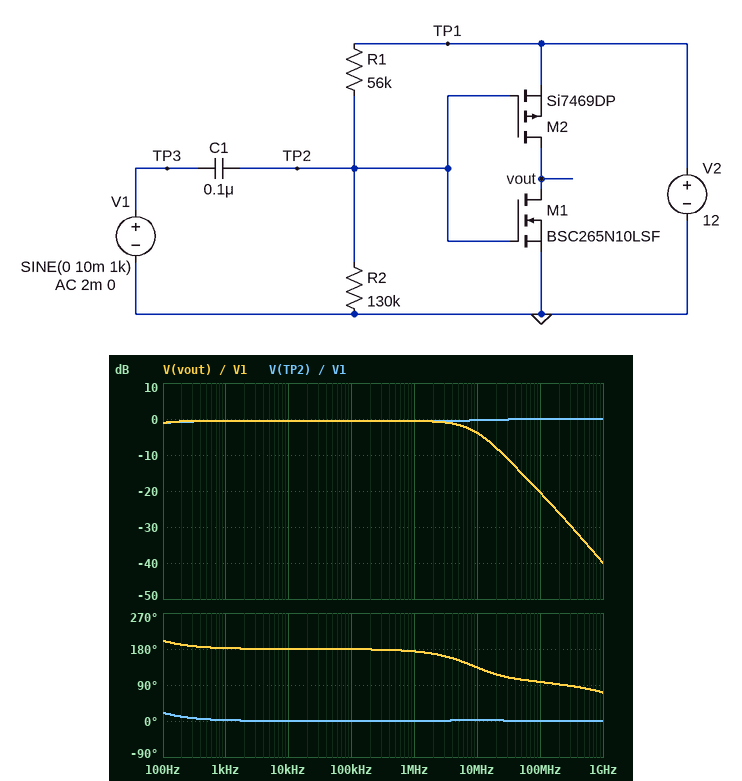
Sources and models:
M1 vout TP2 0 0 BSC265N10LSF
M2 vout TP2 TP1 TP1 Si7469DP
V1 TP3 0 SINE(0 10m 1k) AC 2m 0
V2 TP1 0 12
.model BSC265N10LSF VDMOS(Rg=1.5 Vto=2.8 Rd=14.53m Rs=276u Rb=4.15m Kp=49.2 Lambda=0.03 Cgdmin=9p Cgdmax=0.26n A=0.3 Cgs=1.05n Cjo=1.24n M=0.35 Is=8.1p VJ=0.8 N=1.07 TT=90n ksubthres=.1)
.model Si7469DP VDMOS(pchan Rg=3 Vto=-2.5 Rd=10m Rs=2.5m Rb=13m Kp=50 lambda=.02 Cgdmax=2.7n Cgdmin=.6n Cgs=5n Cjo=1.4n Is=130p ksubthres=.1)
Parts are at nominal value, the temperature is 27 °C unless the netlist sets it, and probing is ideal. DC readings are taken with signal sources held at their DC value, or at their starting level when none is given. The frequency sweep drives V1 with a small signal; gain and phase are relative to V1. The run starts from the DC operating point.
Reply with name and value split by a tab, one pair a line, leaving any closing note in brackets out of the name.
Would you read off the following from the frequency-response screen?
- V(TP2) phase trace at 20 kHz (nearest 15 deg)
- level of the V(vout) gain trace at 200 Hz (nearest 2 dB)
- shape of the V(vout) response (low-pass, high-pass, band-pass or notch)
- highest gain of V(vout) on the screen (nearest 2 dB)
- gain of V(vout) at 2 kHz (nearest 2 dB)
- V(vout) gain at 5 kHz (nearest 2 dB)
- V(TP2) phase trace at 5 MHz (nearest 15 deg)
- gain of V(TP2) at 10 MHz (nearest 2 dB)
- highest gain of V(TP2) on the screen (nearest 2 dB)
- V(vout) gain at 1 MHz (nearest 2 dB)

V(TP2) phase trace at 20 kHz	0 deg
level of the V(vout) gain trace at 200 Hz	0 dB
shape of the V(vout) response	low-pass
highest gain of V(vout) on the screen	0 dB
gain of V(vout) at 2 kHz	0 dB
V(vout) gain at 5 kHz	0 dB
V(TP2) phase trace at 5 MHz	0 deg
gain of V(TP2) at 10 MHz	0 dB
highest gain of V(TP2) on the screen	0 dB
V(vout) gain at 1 MHz	0 dB
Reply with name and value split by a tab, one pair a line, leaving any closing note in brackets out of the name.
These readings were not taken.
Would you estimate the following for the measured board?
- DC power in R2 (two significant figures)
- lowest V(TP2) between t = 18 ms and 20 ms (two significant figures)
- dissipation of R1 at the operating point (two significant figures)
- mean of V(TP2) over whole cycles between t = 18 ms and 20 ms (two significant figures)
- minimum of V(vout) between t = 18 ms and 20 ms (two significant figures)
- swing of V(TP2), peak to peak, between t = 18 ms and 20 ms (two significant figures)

DC power in R2	540 µW
lowest V(TP2) between t = 18 ms and 20 ms	8.4 V
dissipation of R1 at the operating point	230 µW
mean of V(TP2) over whole cycles between t = 18 ms and 20 ms	8.4 V
minimum of V(vout) between t = 18 ms and 20 ms	590 mV
swing of V(TP2), peak to peak, between t = 18 ms and 20 ms	19 mV
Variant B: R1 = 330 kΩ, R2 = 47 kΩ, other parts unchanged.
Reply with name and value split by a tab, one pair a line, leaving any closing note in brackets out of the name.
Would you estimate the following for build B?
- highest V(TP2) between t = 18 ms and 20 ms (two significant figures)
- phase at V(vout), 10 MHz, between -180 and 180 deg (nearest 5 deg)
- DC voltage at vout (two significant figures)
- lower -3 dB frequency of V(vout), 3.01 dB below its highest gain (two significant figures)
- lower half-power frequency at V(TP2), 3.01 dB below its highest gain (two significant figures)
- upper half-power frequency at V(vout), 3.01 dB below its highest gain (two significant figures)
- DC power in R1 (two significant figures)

highest V(TP2) between t = 18 ms and 20 ms	1.5 V
phase at V(vout), 10 MHz, between -180 and 180 deg	40 deg
DC voltage at vout	12 V
lower -3 dB frequency of V(vout), 3.01 dB below its highest gain	15 MHz
lower half-power frequency at V(TP2), 3.01 dB below its highest gain	43 Hz
upper half-power frequency at V(vout), 3.01 dB below its highest gain	4.5 GHz
DC power in R1	330 µW
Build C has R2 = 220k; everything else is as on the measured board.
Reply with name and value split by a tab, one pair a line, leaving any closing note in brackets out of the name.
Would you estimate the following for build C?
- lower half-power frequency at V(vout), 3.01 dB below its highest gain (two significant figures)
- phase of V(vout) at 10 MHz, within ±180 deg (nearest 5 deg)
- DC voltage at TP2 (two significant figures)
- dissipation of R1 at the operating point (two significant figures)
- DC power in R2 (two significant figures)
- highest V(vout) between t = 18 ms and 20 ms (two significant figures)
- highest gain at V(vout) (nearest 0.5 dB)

lower half-power frequency at V(vout), 3.01 dB below its highest gain	33 Hz
phase of V(vout) at 10 MHz, within ±180 deg	130 deg
DC voltage at TP2	9.6 V
dissipation of R1 at the operating point	110 µW
DC power in R2	420 µW
highest V(vout) between t = 18 ms and 20 ms	1.1 mV
highest gain at V(vout)	-36.5 dB
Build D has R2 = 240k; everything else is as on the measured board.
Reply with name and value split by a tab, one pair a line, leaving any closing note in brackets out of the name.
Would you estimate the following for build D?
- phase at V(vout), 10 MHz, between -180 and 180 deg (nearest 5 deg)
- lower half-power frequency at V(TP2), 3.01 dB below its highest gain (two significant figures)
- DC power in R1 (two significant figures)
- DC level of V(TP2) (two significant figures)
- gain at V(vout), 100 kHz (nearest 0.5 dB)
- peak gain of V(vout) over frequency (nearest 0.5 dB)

phase at V(vout), 10 MHz, between -180 and 180 deg	95 deg
lower half-power frequency at V(TP2), 3.01 dB below its highest gain	38 Hz
DC power in R1	92 µW
DC level of V(TP2)	9.7 V
gain at V(vout), 100 kHz	-61.0 dB
peak gain of V(vout) over frequency	-58.0 dB
